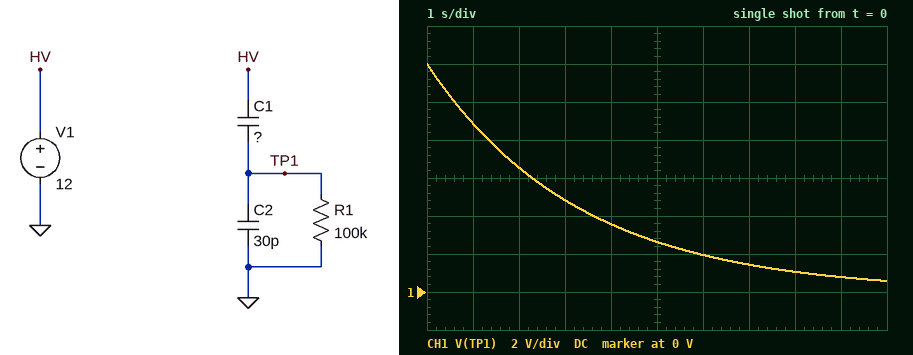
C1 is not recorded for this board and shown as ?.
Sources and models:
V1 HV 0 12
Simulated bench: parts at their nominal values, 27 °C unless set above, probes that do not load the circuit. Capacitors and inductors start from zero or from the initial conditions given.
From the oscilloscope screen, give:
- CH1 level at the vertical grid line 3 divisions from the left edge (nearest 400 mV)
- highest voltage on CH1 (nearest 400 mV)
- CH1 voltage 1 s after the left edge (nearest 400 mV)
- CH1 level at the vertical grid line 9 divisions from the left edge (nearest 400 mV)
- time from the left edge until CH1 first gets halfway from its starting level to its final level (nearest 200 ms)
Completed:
4.8 V
12.0 V
8.8 V
800 mV
2.2 s
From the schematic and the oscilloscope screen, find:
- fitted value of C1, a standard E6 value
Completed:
33 µF
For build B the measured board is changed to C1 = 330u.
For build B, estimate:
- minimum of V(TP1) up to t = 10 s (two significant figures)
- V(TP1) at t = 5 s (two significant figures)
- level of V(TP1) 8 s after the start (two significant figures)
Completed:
8.9 V
10 V
9.4 V
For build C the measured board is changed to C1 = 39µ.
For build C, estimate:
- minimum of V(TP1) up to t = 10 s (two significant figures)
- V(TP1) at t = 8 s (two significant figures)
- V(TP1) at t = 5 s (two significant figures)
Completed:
920 mV
1.5 V
3.3 V
